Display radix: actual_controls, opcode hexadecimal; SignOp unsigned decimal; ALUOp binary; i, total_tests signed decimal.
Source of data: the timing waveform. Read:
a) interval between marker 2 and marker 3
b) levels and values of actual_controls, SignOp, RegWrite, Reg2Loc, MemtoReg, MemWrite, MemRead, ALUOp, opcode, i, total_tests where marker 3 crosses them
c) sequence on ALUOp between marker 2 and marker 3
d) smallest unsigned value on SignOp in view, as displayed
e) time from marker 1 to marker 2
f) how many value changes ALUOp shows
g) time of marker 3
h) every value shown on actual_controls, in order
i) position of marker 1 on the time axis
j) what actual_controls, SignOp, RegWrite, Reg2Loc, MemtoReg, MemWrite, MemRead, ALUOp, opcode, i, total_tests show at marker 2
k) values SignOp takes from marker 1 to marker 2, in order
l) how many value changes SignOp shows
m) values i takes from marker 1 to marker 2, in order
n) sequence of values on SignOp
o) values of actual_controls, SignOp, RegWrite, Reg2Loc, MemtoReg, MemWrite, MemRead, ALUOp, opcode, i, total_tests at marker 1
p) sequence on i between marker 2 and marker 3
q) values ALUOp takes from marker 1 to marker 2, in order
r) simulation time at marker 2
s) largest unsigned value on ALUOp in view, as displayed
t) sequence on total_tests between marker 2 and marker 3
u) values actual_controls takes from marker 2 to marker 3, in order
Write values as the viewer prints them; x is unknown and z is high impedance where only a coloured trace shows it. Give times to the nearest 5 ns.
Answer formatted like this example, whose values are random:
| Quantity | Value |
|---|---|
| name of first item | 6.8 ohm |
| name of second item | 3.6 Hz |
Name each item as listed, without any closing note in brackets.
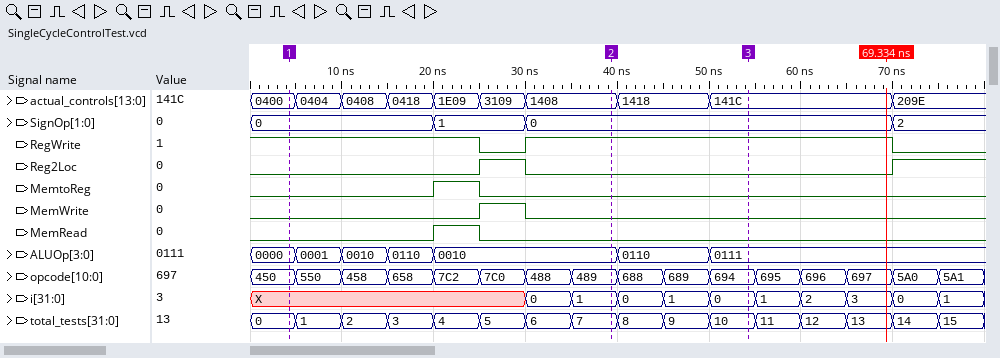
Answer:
| Quantity | Value |
|---|---|
| interval between marker 2 and marker 3 | 15 ns |
| levels and values of actual_controls, SignOp, RegWrite, Reg2Loc, MemtoReg, MemWrite, MemRead, ALUOp, opcode, i, total_tests where marker 3 crosses them | actual_controls=141C, SignOp=0, RegWrite=1, Reg2Loc=0, MemtoReg=0, MemWrite=0, MemRead=0, ALUOp=0111, opcode=694, i=0, total_tests=10 |
| sequence on ALUOp between marker 2 and marker 3 | 0010, 0110, 0111 |
| smallest unsigned value on SignOp in view, as displayed | 0 |
| time from marker 1 to marker 2 | 35 ns |
| how many value changes ALUOp shows | 6 |
| time of marker 3 | 55 ns |
| every value shown on actual_controls, in order | 0400, 0404, 0408, 0418, 1E09, 3109, 1408, 1418, 141C, 209E |
| position of marker 1 on the time axis | 5 ns |
| what actual_controls, SignOp, RegWrite, Reg2Loc, MemtoReg, MemWrite, MemRead, ALUOp, opcode, i, total_tests show at marker 2 | actual_controls=1408, SignOp=0, RegWrite=1, Reg2Loc=0, MemtoReg=0, MemWrite=0, MemRead=0, ALUOp=0010, opcode=489, i=1, total_tests=7 |
| values SignOp takes from marker 1 to marker 2, in order | 0, 1, 0 |
| how many value changes SignOp shows | 3 |
| values i takes from marker 1 to marker 2, in order | X, 0, 1 |
| sequence of values on SignOp | 0, 1, 0, 2 |
| values of actual_controls, SignOp, RegWrite, Reg2Loc, MemtoReg, MemWrite, MemRead, ALUOp, opcode, i, total_tests at marker 1 | actual_controls=0400, SignOp=0, RegWrite=1, Reg2Loc=0, MemtoReg=0, MemWrite=0, MemRead=0, ALUOp=0000, opcode=450, i=X, total_tests=0 |
| sequence on i between marker 2 and marker 3 | 1, 0, 1, 0 |
| values ALUOp takes from marker 1 to marker 2, in order | 0000, 0001, 0010, 0110, 0010 |
| simulation time at marker 2 | 40 ns |
| largest unsigned value on ALUOp in view, as displayed | 0111 |
| sequence on total_tests between marker 2 and marker 3 | 7, 8, 9, 10 |
| values actual_controls takes from marker 2 to marker 3, in order | 1408, 1418, 141C |
